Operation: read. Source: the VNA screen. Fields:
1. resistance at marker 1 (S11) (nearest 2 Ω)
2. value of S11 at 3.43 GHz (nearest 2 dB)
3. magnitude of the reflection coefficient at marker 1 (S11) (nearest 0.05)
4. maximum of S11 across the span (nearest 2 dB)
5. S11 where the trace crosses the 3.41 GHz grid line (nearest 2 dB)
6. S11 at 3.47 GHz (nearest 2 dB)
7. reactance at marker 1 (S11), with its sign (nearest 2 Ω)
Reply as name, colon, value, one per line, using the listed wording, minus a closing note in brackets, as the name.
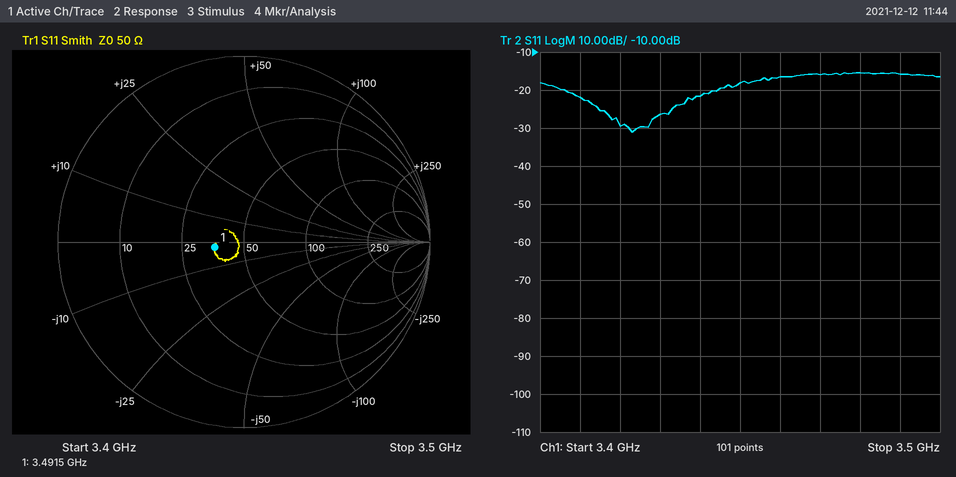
resistance at marker 1 (S11): 36 Ω
value of S11 at 3.43 GHz: -26 dB
magnitude of the reflection coefficient at marker 1 (S11): 0.15
maximum of S11 across the span: -16 dB
S11 where the trace crosses the 3.41 GHz grid line: -22 dB
S11 at 3.47 GHz: -16 dB
reactance at marker 1 (S11), with its sign: -2 Ω
